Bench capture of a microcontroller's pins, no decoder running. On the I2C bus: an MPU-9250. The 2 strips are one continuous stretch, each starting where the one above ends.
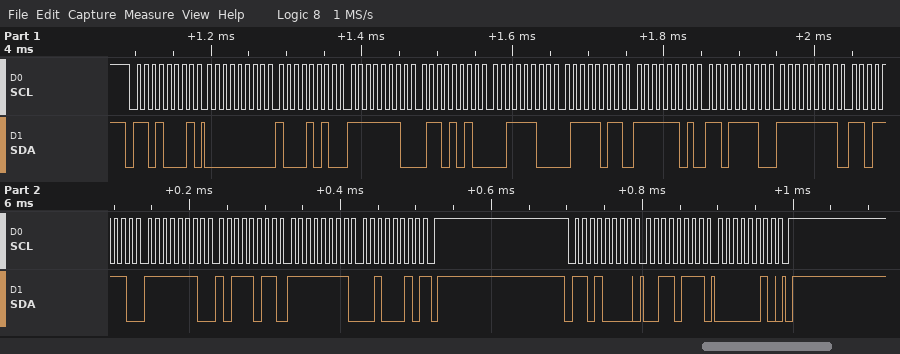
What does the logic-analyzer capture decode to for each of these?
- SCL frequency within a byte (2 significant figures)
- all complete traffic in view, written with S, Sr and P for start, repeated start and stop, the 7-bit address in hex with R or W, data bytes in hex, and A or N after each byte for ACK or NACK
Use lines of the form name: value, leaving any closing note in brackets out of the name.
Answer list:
SCL frequency within a byte: 100 kHz
all complete traffic in view, written with S, Sr and P for start, repeated start and stop, the 7-bit address in hex with R or W, data bytes in hex, and A or N after each byte for ACK or NACK: S 68R A 00 A 8A A FE A 6A A 3C A 7B A FD A DE A FF A DE A FE A BB A FF A 22 N P S 68W A 37 A 02 A P
